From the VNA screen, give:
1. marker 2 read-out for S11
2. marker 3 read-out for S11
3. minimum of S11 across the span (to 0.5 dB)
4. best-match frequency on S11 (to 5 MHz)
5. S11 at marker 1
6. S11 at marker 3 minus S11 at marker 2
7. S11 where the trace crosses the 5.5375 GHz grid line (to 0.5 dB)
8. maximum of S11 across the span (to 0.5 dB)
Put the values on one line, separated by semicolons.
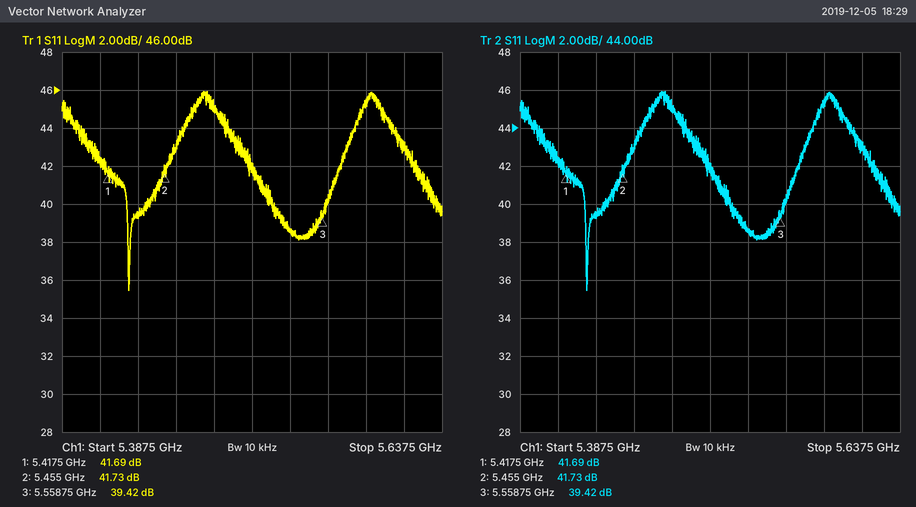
41.73 dB; 39.42 dB; 35.5 dB; 5.430 GHz; 41.69 dB; -2.31 dB; 38.5 dB; 46.0 dB
